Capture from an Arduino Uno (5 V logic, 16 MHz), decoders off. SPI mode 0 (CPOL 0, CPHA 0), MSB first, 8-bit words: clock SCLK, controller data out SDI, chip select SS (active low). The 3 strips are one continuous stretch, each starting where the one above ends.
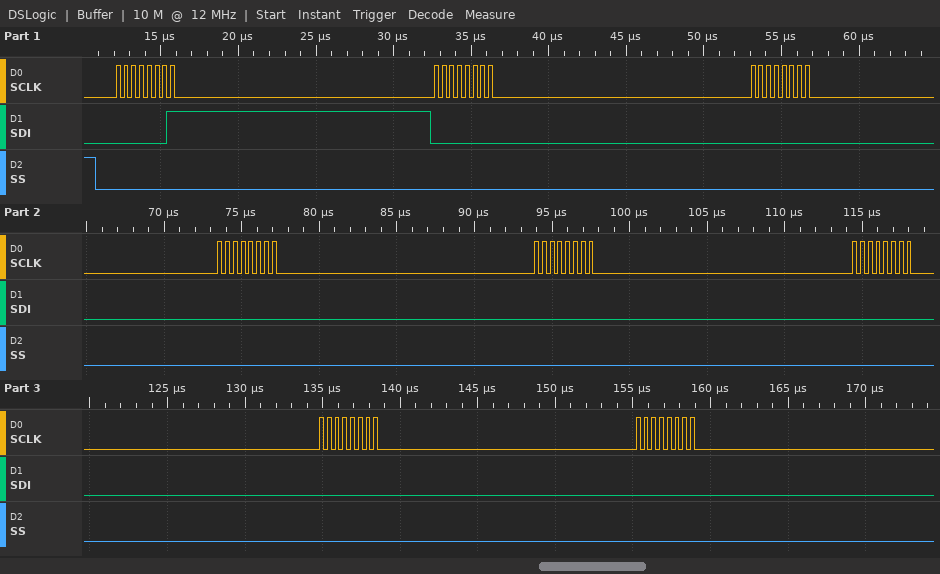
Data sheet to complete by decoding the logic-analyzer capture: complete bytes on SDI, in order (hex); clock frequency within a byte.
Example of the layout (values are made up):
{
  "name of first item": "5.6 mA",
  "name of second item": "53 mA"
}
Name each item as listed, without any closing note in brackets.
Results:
{
  "complete bytes on SDI, in order": "0x01 0x00 0x00 0x00 0x00 0x00 0x00 0x00",
  "clock frequency within a byte": "2 MHz"
}
